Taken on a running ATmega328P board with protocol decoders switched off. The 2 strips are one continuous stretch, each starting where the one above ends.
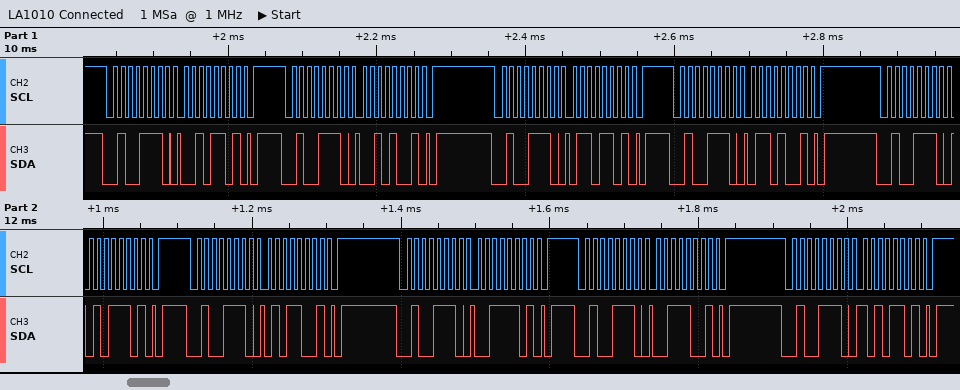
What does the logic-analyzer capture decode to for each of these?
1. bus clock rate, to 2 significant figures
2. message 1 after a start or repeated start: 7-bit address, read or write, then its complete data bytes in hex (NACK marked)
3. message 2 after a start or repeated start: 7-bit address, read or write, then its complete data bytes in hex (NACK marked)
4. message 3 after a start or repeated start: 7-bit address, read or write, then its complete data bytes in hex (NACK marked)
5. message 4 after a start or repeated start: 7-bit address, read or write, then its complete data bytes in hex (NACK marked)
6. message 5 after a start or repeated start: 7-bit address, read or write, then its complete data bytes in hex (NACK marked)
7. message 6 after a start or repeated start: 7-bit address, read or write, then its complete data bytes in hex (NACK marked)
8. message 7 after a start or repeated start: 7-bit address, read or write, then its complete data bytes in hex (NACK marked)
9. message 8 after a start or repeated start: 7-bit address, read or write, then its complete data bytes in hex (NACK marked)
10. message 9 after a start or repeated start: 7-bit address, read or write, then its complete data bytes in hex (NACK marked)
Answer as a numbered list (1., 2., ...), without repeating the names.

1. 100 kHz
2. 0x27 write: 2D
3. 0x27 write: 29
4. 0x27 write: 6D
5. 0x27 write: 69
6. 0x27 write: 5D
7. 0x27 write: 59
8. 0x27 write: 3D
9. 0x27 write: 39
10. 0x27 write: AD
